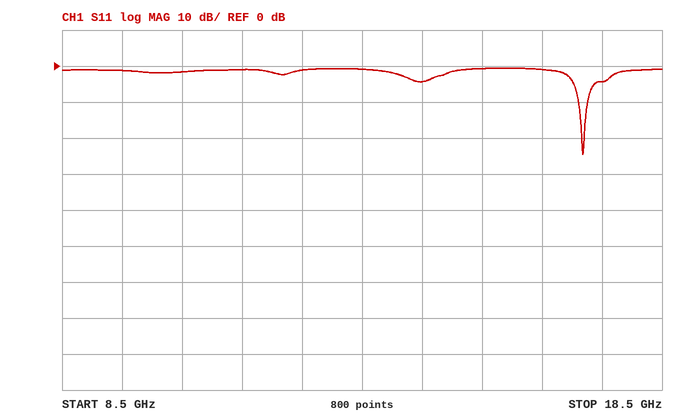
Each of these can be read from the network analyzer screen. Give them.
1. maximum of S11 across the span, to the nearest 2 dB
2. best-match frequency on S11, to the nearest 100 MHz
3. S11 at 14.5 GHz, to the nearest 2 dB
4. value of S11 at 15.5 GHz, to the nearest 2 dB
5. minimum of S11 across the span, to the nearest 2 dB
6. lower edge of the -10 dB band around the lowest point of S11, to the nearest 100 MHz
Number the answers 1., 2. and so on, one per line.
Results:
1. 0 dB
2. 17.2 GHz
3. -4 dB
4. 0 dB
5. -24 dB
6. 17.1 GHz
